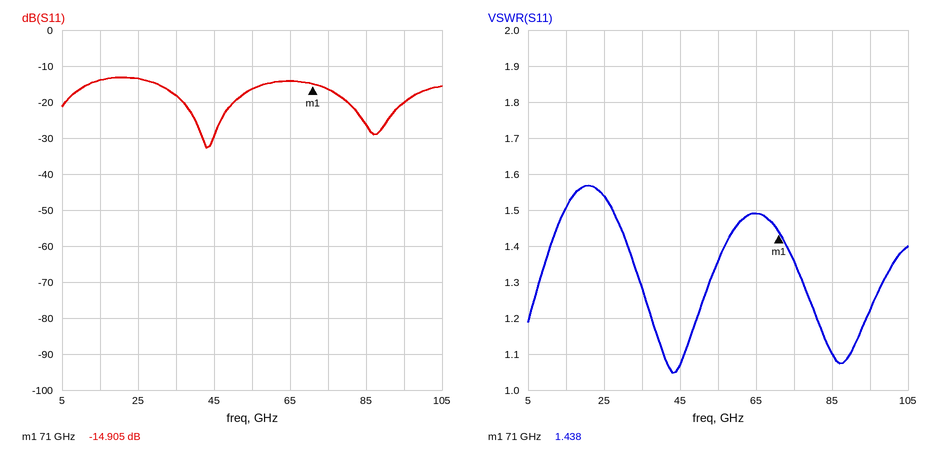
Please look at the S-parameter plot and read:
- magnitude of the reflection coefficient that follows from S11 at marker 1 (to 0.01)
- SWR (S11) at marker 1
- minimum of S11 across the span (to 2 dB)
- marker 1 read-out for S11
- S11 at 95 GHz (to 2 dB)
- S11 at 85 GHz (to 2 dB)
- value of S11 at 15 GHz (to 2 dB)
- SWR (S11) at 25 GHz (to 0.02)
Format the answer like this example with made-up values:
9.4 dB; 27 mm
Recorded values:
0.18; 1.438; -32 dB; -14.905 dB; -20 dB; -26 dB; -14 dB; 1.54
